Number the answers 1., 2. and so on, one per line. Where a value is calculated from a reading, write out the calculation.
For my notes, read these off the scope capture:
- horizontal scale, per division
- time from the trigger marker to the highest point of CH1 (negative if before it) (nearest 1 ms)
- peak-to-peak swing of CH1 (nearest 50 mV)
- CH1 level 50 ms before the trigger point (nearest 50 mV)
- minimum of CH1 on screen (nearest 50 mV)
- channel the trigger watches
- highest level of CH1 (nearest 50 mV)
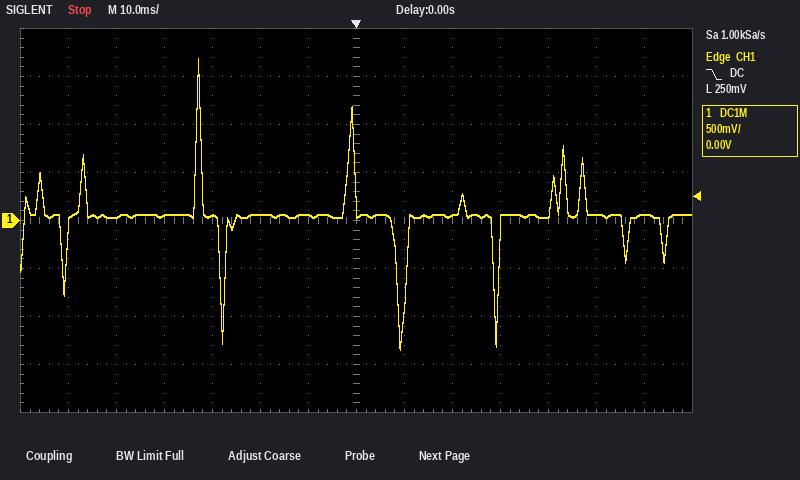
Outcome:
1. 10 ms
2. -33 ms
3. 1.70 V − (-1.35 V) = 3.05 V
4. 50 mV
5. -1.35 V
6. CH1
7. 1.70 V
